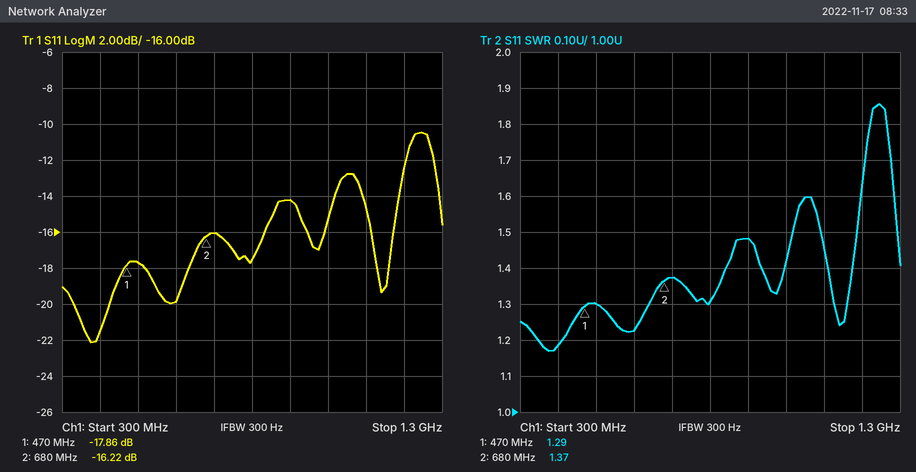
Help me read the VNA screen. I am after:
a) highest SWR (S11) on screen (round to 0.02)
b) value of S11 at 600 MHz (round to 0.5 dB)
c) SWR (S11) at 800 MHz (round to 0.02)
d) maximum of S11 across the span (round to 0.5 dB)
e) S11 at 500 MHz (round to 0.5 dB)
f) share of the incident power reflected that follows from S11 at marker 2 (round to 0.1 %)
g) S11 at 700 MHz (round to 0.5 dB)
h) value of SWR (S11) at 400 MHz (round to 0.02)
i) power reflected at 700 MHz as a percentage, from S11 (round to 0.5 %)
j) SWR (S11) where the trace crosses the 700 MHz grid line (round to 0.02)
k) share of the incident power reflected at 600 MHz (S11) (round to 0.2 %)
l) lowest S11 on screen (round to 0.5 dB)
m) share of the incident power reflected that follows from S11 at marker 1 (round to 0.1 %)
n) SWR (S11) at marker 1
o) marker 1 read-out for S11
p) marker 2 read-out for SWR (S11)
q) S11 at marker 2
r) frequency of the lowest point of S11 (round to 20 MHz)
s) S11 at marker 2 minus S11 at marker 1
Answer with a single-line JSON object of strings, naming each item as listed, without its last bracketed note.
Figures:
{"highest SWR (S11) on screen": "1.86", "value of S11 at 600 MHz": "-20.0 dB", "SWR (S11) at 800 MHz": "1.30", "maximum of S11 across the span": "-10.5 dB", "S11 at 500 MHz": "-17.5 dB", "share of the incident power reflected that follows from S11 at marker 2": "2.4 %", "S11 at 700 MHz": "-16.0 dB", "value of SWR (S11) at 400 MHz": "1.18", "power reflected at 700 MHz as a percentage, from S11": "2.5 %", "SWR (S11) where the trace crosses the 700 MHz grid line": "1.38", "share of the incident power reflected at 600 MHz (S11)": "1.0 %", "lowest S11 on screen": "-22.0 dB", "share of the incident power reflected that follows from S11 at marker 1": "1.6 %", "SWR (S11) at marker 1": "1.29", "marker 1 read-out for S11": "-17.86 dB", "marker 2 read-out for SWR": "1.37", "S11 at marker 2": "-16.22 dB", "frequency of the lowest point of S11": "380 MHz", "S11 at marker 2 minus S11 at marker 1": "1.64 dB"}
